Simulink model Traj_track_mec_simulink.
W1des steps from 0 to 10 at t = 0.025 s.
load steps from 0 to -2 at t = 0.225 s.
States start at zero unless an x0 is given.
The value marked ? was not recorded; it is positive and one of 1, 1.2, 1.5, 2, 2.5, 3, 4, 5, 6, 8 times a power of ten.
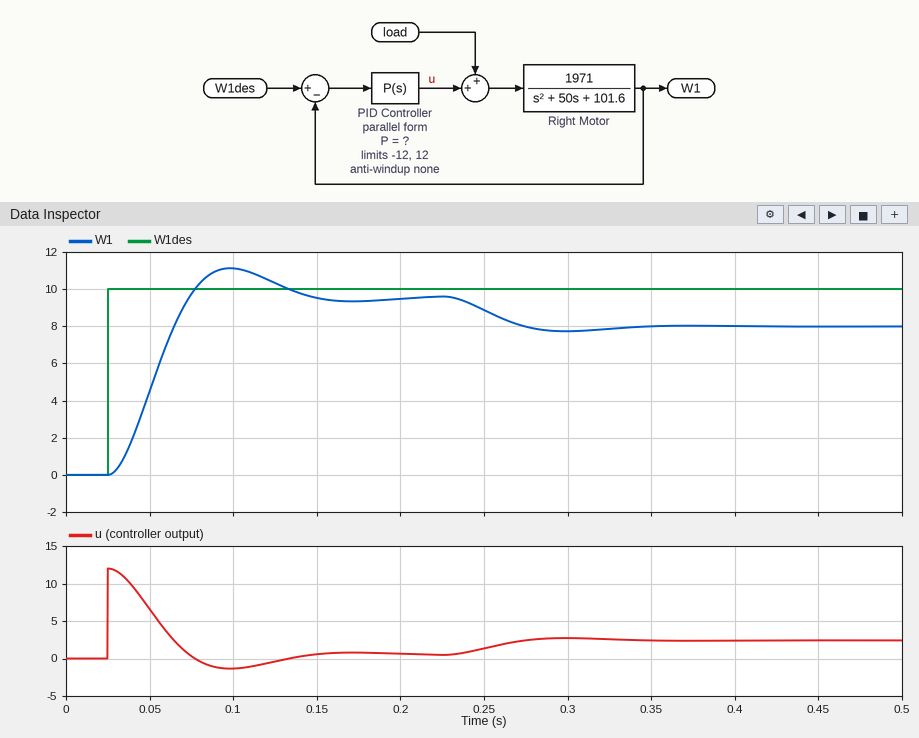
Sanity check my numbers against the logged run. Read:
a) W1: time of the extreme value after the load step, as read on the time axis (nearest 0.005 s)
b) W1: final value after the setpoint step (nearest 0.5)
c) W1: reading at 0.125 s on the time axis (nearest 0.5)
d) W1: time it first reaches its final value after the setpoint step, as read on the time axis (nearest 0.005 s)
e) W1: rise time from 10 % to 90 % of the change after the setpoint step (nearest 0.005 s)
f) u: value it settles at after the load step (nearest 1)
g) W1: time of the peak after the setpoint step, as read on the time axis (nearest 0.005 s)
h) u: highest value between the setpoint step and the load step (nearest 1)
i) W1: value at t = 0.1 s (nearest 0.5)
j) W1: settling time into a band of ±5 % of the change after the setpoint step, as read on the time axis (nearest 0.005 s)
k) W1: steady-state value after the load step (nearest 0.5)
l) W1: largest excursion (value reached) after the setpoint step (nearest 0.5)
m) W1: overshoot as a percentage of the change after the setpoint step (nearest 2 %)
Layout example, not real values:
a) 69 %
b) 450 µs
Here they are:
a) 0.300 s
b) 9.5
c) 10.5
d) 0.075 s
e) 0.035 s
f) 2
g) 0.100 s
h) 12
i) 11.0
j) 0.130 s
k) 8.0
l) 11.0
m) 16 %
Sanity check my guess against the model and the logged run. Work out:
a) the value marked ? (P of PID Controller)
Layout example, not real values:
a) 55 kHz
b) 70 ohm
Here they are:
a) 1.2
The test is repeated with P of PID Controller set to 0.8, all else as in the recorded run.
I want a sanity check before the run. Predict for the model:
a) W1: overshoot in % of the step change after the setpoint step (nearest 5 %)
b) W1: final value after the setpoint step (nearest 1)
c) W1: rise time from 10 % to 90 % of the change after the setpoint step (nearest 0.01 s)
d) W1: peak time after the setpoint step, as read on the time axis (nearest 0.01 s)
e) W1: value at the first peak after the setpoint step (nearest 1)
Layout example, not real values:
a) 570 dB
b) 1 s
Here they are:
a) 10 %
b) 9
c) 0.05 s
d) 0.12 s
e) 10
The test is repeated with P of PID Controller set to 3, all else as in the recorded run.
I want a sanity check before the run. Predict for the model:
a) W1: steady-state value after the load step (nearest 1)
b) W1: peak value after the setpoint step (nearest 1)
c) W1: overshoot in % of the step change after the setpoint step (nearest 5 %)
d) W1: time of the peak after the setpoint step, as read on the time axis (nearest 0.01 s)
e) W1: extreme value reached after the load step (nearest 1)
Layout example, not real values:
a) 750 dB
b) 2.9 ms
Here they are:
a) 9
b) 12
c) 25 %
d) 0.08 s
e) 9
